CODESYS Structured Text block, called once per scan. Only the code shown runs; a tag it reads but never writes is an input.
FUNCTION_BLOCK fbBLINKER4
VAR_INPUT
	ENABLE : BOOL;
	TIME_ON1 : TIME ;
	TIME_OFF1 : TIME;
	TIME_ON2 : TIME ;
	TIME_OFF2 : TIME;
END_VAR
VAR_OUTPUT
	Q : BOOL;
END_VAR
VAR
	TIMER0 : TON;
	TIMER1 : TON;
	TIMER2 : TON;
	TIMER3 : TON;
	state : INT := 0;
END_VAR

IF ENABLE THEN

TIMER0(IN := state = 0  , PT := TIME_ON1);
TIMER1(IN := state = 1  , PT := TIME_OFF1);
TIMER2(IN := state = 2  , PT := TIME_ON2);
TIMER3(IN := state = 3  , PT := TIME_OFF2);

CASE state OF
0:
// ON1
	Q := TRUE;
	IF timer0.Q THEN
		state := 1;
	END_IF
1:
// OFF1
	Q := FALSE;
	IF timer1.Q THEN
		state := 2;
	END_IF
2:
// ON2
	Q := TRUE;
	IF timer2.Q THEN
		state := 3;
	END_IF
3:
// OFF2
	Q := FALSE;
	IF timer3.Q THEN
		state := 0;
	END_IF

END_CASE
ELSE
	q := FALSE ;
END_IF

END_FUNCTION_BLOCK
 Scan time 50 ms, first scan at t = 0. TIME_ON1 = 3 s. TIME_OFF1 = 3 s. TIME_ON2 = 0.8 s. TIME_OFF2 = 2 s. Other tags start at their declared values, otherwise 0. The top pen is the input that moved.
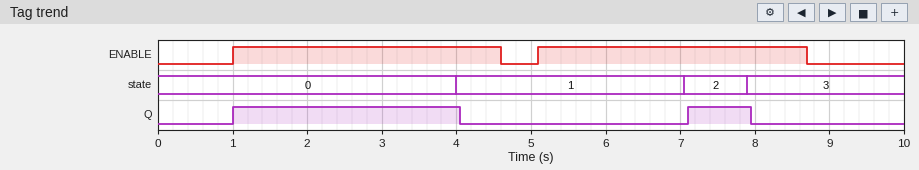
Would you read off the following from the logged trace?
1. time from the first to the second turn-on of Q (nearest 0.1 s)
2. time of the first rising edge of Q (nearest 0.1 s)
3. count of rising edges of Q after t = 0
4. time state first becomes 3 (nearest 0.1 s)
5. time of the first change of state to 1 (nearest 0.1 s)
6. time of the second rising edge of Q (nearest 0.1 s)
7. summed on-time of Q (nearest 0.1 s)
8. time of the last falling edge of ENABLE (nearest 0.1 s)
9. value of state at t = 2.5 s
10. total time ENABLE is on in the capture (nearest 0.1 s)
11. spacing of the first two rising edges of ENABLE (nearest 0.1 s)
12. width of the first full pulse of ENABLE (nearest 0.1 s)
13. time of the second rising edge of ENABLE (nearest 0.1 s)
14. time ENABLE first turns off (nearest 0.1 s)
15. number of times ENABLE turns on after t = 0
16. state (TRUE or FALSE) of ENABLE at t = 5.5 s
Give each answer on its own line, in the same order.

6.1 s
1.0 s
2
7.9 s
4.0 s
7.1 s
3.9 s
8.7 s
0
7.2 s
4.1 s
3.6 s
5.1 s
4.6 s
2
TRUE
